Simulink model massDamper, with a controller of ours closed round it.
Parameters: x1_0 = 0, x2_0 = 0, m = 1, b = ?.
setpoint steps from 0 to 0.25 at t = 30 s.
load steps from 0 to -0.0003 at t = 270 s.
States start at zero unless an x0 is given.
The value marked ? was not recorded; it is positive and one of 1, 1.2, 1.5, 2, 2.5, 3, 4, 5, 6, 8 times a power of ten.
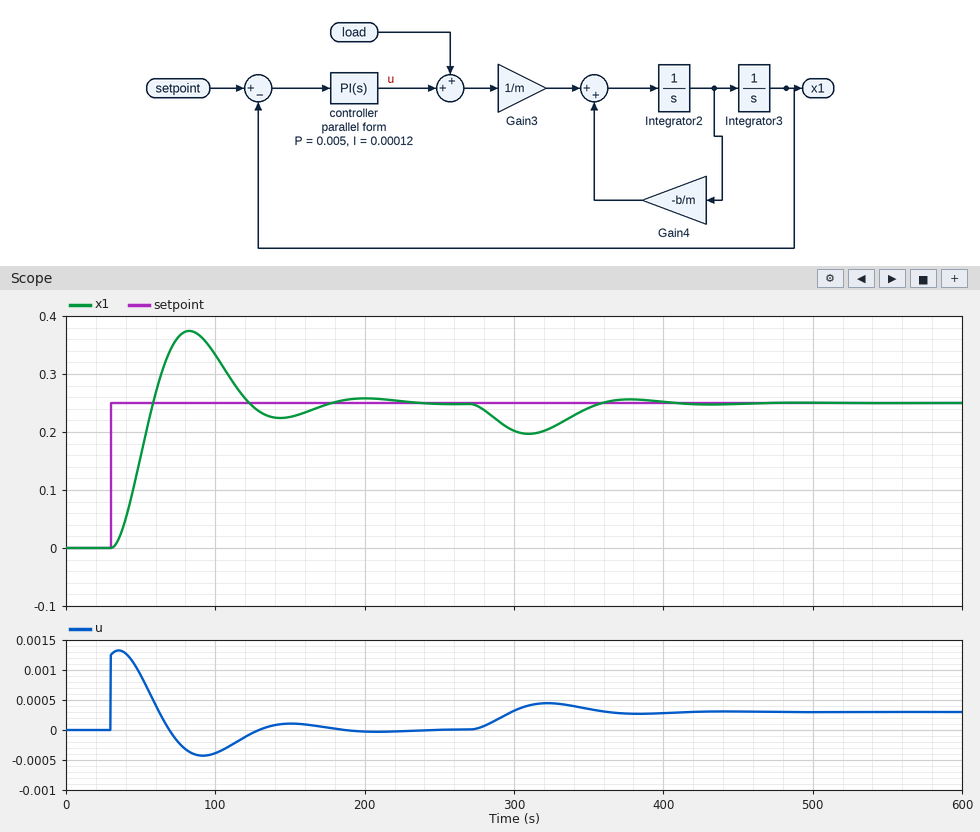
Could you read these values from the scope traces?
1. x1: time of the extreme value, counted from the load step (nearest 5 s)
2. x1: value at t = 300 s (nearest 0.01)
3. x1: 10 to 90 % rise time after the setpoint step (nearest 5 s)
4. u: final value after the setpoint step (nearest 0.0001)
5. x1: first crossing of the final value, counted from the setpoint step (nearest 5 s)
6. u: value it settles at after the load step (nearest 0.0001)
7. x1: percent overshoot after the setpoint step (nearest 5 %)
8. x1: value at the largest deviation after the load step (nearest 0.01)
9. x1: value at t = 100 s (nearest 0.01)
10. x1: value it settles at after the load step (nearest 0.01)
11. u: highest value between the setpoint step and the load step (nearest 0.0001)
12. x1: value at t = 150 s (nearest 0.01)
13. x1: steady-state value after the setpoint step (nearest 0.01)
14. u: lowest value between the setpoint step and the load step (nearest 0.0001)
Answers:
40 s
0.20
20 s
0.0000
30 s
0.0003
50 %
0.20
0.33
0.25
0.0013
0.23
0.25
-0.0004
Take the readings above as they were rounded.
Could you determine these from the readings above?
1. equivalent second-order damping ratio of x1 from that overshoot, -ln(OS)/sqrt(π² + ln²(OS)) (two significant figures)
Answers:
0.22
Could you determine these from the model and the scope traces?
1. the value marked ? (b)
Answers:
0.08
